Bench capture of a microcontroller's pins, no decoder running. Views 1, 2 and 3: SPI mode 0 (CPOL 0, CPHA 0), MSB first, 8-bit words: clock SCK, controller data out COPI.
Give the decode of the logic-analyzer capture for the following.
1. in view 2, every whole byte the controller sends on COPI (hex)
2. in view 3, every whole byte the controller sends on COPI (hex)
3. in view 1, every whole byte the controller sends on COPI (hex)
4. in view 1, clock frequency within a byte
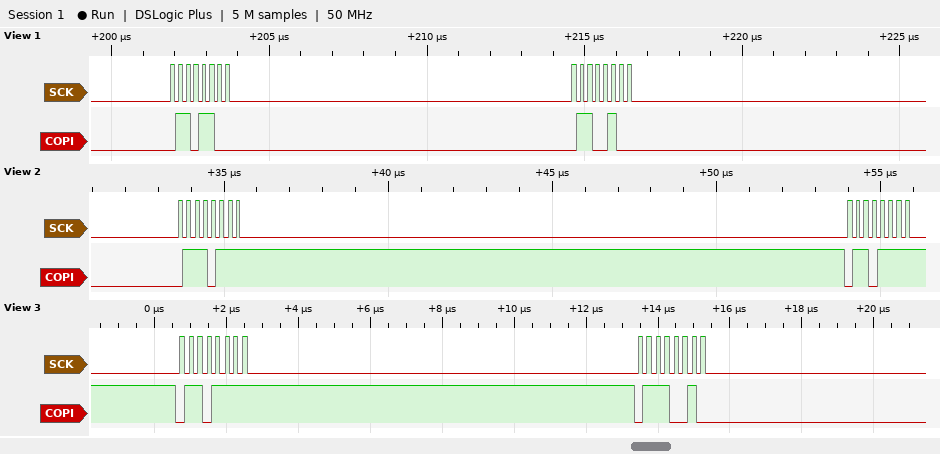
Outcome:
77 6F
0x6F 0x72
6C 64
4 MHz
